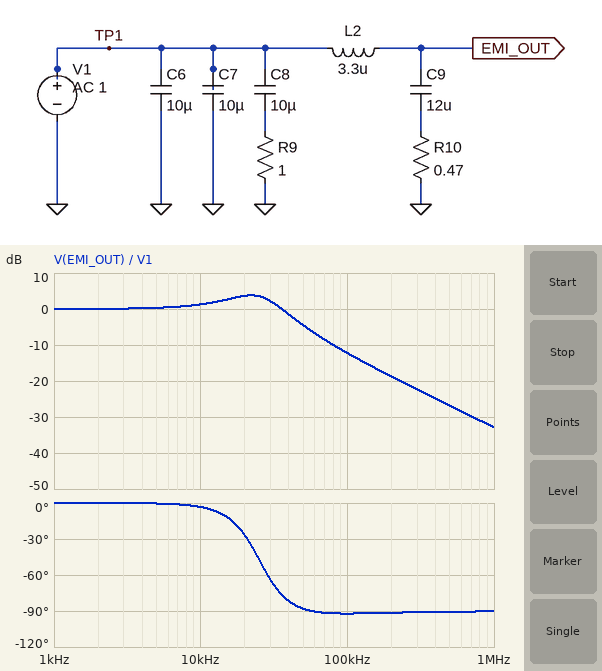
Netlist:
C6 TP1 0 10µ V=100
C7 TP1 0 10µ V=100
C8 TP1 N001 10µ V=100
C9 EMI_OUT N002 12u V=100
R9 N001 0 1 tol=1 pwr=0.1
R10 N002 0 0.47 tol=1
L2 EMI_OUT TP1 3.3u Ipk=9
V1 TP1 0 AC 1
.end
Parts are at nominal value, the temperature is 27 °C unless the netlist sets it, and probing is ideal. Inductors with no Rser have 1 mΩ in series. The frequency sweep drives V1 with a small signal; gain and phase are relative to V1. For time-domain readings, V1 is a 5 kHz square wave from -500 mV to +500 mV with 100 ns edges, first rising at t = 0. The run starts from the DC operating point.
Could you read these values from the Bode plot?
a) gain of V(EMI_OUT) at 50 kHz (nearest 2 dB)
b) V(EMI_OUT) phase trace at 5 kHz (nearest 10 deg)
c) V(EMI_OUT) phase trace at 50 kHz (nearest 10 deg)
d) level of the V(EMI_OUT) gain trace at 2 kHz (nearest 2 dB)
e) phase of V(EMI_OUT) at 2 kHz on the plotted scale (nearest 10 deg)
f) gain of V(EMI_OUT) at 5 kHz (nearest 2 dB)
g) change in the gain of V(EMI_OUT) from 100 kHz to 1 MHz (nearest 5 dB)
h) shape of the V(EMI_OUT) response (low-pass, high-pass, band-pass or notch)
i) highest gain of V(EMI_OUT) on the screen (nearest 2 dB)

-4 dB
0 deg
-90 deg
0 dB
0 deg
0 dB
-20 dB
low-pass
4 dB
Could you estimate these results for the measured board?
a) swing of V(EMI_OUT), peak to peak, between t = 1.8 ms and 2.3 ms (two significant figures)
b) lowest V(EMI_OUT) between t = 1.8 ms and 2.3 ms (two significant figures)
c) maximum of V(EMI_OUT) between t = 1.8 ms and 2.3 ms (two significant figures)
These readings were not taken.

1.7 V
-830 mV
830 mV
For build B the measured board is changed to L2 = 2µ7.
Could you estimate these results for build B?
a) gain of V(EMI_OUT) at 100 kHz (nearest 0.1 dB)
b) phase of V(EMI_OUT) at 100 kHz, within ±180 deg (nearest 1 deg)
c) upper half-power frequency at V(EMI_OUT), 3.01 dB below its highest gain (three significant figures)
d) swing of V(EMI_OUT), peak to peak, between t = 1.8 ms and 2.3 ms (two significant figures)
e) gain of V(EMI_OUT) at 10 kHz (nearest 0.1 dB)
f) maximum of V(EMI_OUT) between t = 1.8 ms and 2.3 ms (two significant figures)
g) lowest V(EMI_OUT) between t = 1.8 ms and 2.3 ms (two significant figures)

-10.5 dB
-89 deg
38.3 kHz
1.6 V
1.0 dB
800 mV
-800 mV
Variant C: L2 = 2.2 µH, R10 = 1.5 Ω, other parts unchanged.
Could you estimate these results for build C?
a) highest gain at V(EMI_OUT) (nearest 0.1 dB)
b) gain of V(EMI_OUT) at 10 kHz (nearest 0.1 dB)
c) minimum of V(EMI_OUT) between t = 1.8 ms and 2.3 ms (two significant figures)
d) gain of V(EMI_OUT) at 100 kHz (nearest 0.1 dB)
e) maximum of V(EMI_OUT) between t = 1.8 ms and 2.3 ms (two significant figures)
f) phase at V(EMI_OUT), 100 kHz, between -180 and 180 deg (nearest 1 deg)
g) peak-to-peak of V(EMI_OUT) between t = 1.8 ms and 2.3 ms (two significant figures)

0.5 dB
0.4 dB
-560 mV
-2.3 dB
560 mV
-45 deg
1.1 V
